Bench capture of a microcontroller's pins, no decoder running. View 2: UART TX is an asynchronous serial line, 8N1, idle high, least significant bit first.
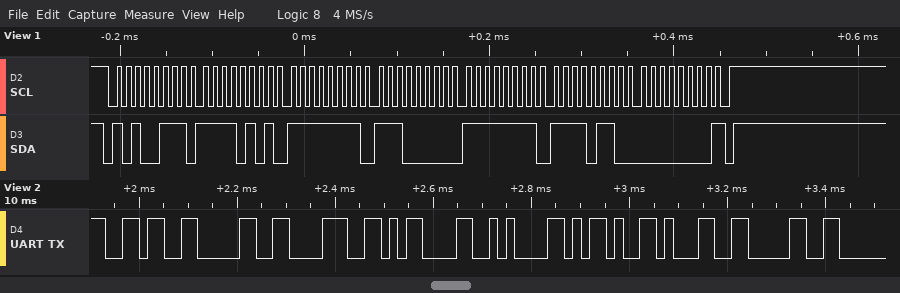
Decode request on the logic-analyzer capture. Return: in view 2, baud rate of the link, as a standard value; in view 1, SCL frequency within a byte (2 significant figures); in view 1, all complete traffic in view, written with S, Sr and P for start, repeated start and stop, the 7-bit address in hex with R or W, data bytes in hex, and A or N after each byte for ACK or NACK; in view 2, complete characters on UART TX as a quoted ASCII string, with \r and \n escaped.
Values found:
57600 baud
100 kHz
S 53R A F5 A FF A E0 A FF A F6 A 00 N P
"608\r\n-10"
